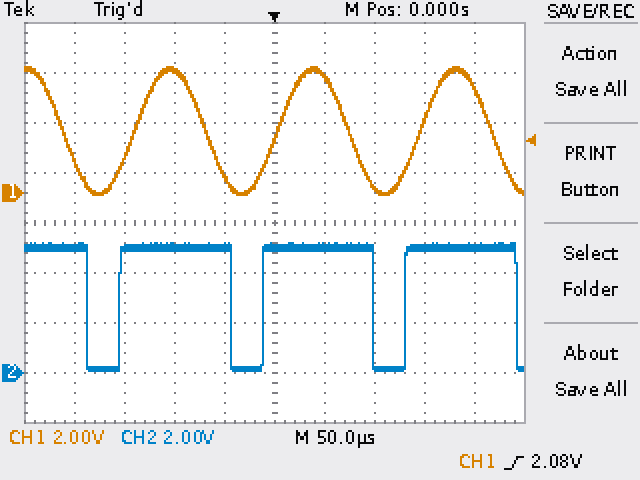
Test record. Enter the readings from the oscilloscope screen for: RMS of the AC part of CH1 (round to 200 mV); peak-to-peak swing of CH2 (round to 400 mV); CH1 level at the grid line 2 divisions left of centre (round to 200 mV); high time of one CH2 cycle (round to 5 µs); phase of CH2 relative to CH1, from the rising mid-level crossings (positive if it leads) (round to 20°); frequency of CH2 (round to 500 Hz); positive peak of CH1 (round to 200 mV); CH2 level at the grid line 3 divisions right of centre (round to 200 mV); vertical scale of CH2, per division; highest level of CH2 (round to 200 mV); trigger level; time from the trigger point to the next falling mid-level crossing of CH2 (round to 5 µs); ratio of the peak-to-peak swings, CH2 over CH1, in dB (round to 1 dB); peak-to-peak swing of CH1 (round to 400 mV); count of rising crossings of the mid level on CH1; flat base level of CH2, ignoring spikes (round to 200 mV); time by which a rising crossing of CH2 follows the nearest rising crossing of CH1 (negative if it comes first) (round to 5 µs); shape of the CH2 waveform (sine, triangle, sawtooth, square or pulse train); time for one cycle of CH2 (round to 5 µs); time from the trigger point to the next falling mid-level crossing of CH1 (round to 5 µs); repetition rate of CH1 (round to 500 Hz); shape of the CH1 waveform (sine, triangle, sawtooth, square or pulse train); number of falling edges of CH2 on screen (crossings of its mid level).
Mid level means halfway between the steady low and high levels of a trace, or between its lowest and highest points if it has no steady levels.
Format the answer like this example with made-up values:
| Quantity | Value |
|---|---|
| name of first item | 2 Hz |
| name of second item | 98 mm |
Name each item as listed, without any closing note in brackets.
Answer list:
| Quantity | Value |
|---|---|
| RMS of the AC part of CH1 | 1.8 V |
| peak-to-peak swing of CH2 | 5.2 V |
| CH1 level at the grid line 2 divisions left of centre | 4.8 V |
| high time of one CH2 cycle | 110 µs |
| phase of CH2 relative to CH1, from the rising mid-level crossings (positive if it leads) | +40° |
| frequency of CH2 | 7.0 kHz |
| positive peak of CH1 | 5.0 V |
| CH2 level at the grid line 3 divisions right of centre | 5.0 V |
| vertical scale of CH2, per division | 2 V |
| highest level of CH2 | 5.2 V |
| trigger level | 2.08 V |
| time from the trigger point to the next falling mid-level crossing of CH2 | 100 µs |
| ratio of the peak-to-peak swings, CH2 over CH1, in dB | 0 dB |
| peak-to-peak swing of CH1 | 5.2 V |
| count of rising crossings of the mid level on CH1 | 3 |
| flat base level of CH2, ignoring spikes | 200 mV |
| time by which a rising crossing of CH2 follows the nearest rising crossing of CH1 (negative if it comes first) | -15 µs |
| shape of the CH2 waveform | pulse train |
| time for one cycle of CH2 | 145 µs |
| time from the trigger point to the next falling mid-level crossing of CH1 | 75 µs |
| repetition rate of CH1 | 7.0 kHz |
| shape of the CH1 waveform | sine |
| number of falling edges of CH2 on screen | 4 |
